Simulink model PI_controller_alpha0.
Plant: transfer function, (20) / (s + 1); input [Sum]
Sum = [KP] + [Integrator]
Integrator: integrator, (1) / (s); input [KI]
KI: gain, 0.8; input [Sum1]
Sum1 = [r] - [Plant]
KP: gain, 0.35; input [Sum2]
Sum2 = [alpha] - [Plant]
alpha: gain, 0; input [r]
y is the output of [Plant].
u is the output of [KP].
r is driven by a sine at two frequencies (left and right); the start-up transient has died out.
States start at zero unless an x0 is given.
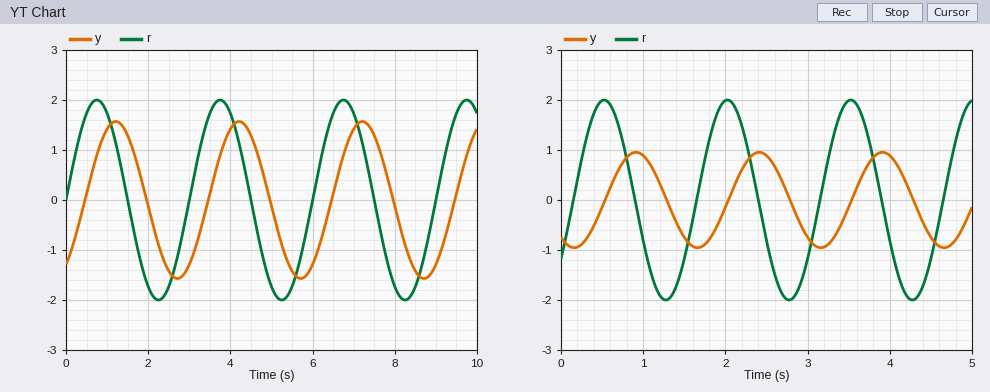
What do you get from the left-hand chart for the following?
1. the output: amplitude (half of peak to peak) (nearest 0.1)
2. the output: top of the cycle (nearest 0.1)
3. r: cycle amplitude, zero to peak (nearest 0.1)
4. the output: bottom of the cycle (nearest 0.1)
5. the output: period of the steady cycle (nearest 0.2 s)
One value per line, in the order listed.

1.6
1.6
2.0
-1.6
3.0 s
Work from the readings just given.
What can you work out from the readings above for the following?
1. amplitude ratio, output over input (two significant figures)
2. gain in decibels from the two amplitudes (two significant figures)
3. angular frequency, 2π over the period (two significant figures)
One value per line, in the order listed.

0.80
-1.9 dB
2.1 rad/s
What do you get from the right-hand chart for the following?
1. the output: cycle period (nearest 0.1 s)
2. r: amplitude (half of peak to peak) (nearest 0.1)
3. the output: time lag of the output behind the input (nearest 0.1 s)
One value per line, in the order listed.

1.5 s
2.0
0.4 s
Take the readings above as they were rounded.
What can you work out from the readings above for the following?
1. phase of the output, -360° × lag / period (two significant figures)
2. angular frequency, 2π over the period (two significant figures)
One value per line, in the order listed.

-96°
4.2 rad/s
